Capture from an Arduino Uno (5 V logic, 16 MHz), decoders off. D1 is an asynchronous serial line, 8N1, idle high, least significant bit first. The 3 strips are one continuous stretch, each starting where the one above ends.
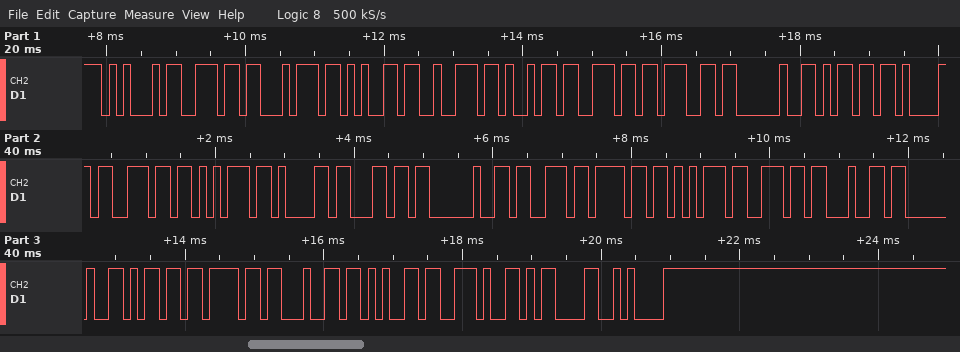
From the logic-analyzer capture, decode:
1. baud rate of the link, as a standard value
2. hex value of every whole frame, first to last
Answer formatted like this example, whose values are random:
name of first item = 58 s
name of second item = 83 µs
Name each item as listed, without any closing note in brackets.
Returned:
baud rate of the link, as a standard value = 9600 baud
hex value of every whole frame, first to last = 45 6E 74 65 72 69 6E 67 20 6D 61 6E 75 61 6C 20 73 6F 75 6E 64 20 6D 6F 64 65 2E 0D 0A
